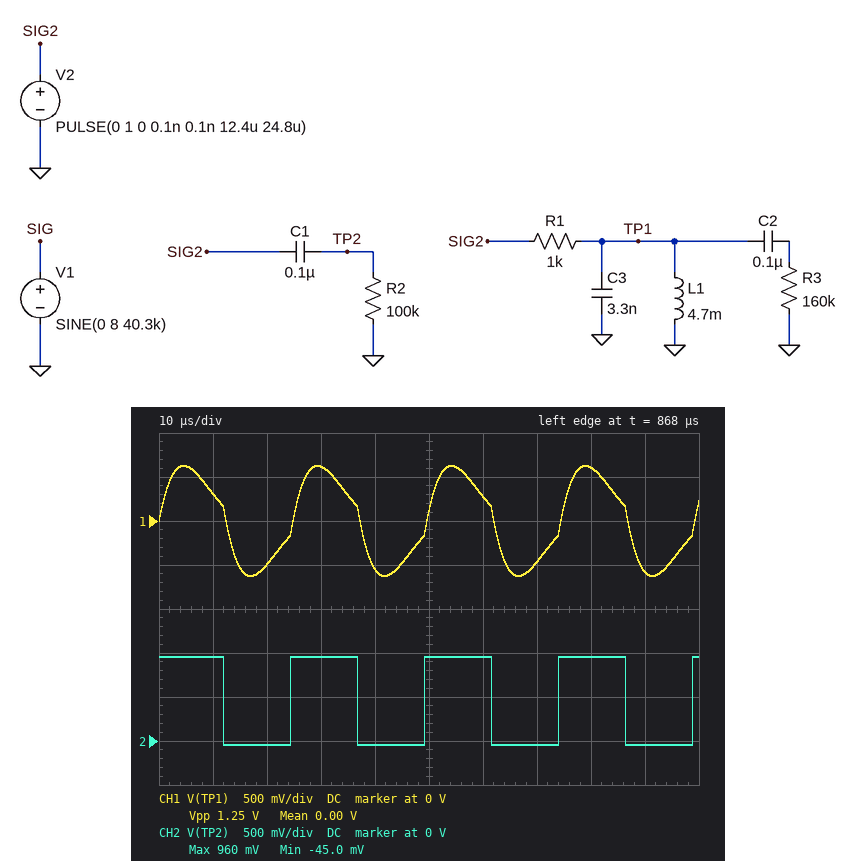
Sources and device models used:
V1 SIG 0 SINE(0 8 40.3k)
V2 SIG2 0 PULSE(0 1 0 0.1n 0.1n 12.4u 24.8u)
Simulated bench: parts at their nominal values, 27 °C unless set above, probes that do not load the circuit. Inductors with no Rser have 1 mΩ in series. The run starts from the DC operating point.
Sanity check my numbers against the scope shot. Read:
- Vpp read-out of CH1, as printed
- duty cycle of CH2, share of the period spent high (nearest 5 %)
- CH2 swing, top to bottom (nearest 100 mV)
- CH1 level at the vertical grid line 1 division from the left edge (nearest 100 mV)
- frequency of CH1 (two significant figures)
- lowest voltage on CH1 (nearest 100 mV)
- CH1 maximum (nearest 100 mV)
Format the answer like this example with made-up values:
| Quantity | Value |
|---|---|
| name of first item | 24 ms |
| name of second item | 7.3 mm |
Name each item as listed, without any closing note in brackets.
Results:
| Quantity | Value |
|---|---|
| Vpp read-out of CH1, as printed | 1.25 V |
| duty cycle of CH2, share of the period spent high | 50 % |
| CH2 swing, top to bottom | 1.0 V |
| CH1 level at the vertical grid line 1 division from the left edge | 300 mV |
| frequency of CH1 | 40 kHz |
| lowest voltage on CH1 | -600 mV |
| CH1 maximum | 600 mV |
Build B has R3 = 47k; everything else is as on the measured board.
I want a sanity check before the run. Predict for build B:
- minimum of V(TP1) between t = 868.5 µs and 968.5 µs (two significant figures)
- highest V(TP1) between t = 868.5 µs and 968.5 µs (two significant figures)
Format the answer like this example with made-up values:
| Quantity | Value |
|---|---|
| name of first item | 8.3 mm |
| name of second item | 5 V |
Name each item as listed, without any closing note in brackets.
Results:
| Quantity | Value |
|---|---|
| minimum of V(TP1) between t = 868.5 µs and 968.5 µs | -620 mV |
| highest V(TP1) between t = 868.5 µs and 968.5 µs | 620 mV |
